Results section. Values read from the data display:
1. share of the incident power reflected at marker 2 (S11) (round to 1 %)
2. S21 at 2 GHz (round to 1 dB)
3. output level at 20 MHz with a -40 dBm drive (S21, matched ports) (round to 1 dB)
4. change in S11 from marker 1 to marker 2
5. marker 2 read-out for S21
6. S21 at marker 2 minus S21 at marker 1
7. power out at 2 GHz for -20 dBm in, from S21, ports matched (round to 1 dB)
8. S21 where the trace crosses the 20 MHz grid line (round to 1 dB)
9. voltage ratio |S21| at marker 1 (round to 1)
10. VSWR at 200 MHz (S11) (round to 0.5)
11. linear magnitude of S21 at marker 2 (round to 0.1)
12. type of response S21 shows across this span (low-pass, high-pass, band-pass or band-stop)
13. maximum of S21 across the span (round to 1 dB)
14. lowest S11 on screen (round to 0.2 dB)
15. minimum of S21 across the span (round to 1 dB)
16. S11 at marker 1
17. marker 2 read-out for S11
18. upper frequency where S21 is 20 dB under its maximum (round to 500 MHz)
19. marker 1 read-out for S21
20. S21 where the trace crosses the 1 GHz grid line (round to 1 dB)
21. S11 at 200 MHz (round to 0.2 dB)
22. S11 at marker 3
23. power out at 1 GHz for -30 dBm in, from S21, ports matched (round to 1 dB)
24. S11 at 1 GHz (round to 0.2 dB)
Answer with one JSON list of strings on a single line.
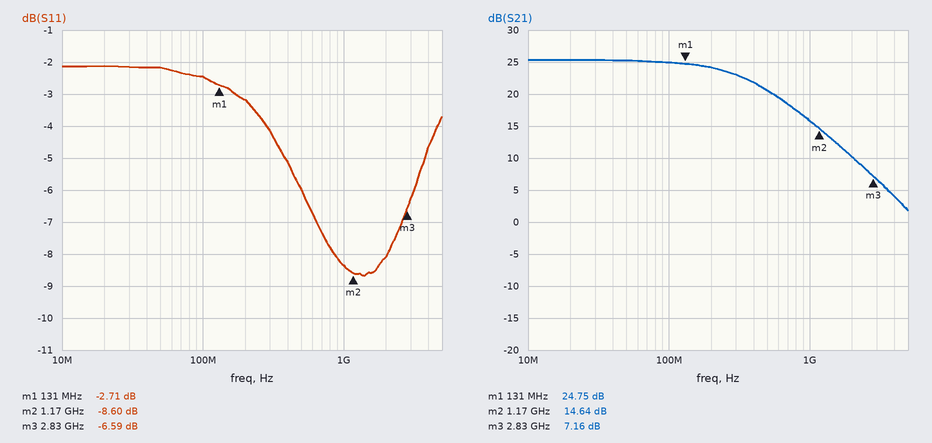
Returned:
["14 %", "10 dB", "-15 dBm", "-5.89 dB", "14.64 dB", "-10.11 dB", "-10 dBm", "25 dB", "17", "5.5", "5.4", "low-pass", "25 dB", "-8.6 dB", "2 dB", "-2.71 dB", "-8.60 dB", "3.5 GHz", "24.75 dB", "16 dB", "-3.2 dB", "-6.59 dB", "-14 dBm", "-8.4 dB"]
